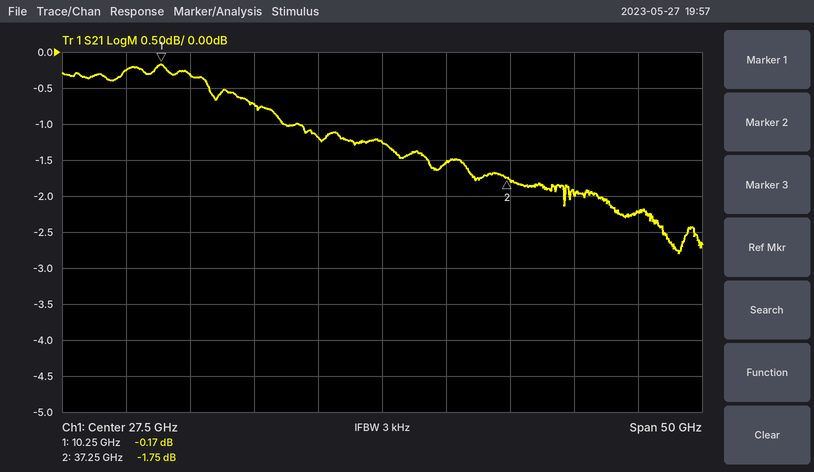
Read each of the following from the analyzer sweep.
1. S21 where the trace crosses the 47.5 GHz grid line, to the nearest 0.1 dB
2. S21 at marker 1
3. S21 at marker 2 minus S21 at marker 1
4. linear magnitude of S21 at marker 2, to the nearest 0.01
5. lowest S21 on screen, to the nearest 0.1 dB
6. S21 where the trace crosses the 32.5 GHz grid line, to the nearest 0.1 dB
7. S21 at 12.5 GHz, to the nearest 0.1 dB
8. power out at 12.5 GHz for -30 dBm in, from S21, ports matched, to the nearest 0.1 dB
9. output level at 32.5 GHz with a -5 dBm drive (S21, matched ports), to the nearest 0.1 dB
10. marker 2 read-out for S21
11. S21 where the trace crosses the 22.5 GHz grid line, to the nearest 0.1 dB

-2.2 dB
-0.17 dB
-1.58 dB
0.82
-2.8 dB
-1.5 dB
-0.3 dB
-30.3 dBm
-6.5 dBm
-1.75 dB
-1.2 dB
